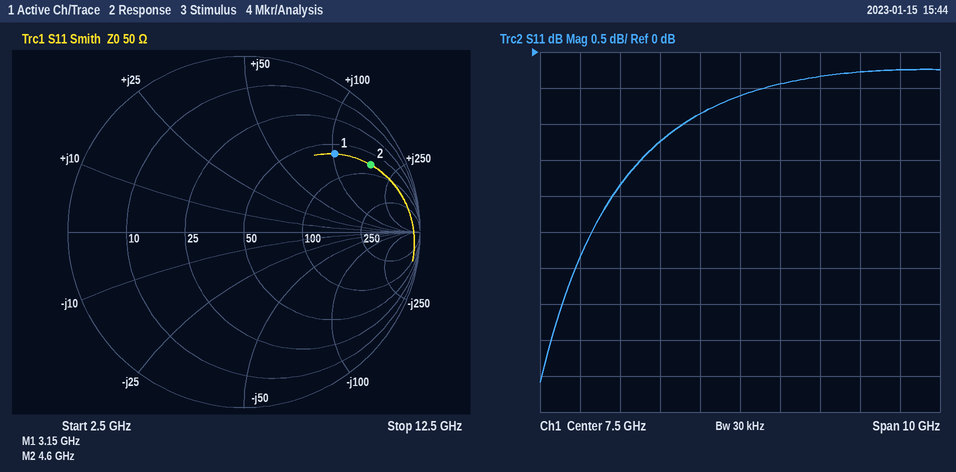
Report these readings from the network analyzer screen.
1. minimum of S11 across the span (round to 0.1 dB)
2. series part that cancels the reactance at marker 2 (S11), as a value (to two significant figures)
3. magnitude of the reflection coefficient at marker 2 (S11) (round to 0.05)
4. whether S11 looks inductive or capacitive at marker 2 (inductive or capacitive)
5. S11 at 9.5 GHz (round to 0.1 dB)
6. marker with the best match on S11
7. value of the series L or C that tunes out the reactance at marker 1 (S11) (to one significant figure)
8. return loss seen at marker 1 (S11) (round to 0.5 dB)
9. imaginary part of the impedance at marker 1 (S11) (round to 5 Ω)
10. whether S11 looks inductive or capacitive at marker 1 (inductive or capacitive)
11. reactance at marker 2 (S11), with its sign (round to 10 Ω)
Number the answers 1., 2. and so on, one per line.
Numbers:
1. -4.6 dB
2. 200 fF
3. 0.80
4. inductive
5. -0.3 dB
6. marker 1
7. 500 fF
8. 3.5 dB
9. +105 Ω
10. inductive
11. +170 Ω
